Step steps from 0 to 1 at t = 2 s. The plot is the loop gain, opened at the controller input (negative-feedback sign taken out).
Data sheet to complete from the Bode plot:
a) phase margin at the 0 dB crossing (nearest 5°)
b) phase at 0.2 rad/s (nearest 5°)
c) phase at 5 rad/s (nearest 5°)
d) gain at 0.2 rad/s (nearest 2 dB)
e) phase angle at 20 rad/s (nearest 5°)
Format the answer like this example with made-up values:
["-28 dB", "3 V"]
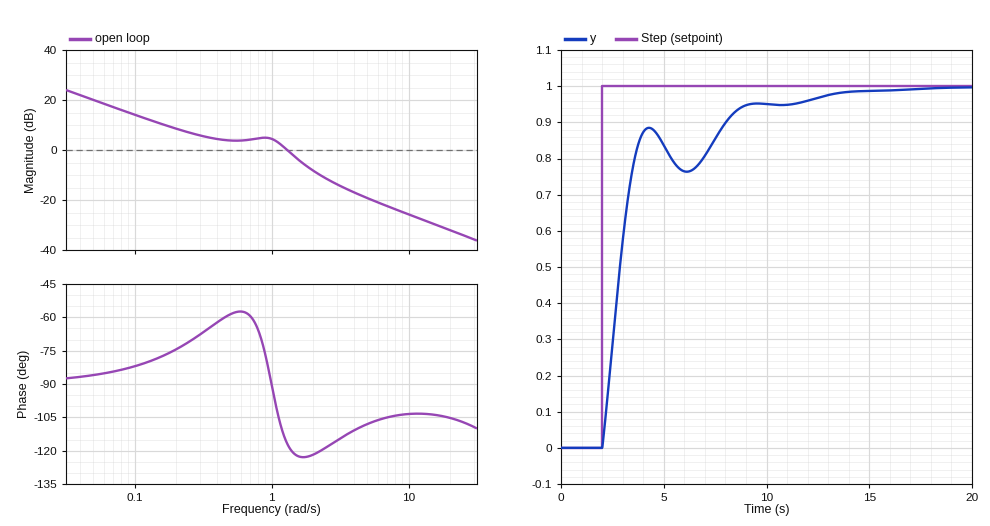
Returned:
["65°", "-75°", "-110°", "8 dB", "-105°"]
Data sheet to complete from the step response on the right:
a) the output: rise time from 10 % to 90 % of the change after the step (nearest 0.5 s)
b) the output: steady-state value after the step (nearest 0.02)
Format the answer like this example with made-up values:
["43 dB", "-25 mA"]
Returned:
["6.0 s", "1.00"]
